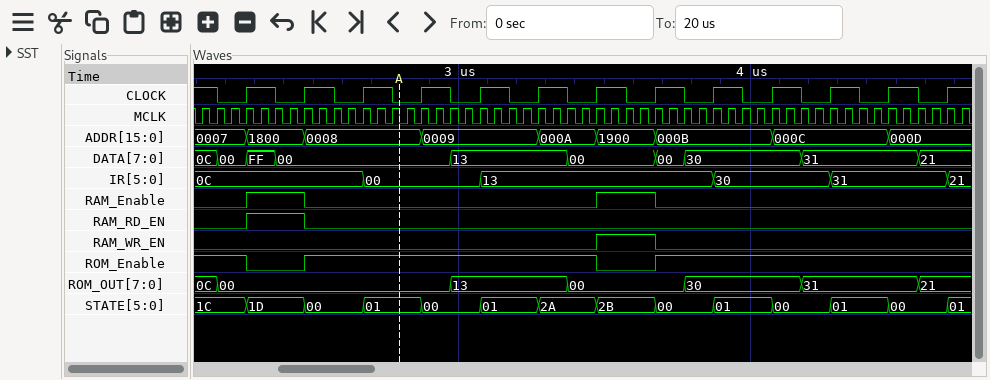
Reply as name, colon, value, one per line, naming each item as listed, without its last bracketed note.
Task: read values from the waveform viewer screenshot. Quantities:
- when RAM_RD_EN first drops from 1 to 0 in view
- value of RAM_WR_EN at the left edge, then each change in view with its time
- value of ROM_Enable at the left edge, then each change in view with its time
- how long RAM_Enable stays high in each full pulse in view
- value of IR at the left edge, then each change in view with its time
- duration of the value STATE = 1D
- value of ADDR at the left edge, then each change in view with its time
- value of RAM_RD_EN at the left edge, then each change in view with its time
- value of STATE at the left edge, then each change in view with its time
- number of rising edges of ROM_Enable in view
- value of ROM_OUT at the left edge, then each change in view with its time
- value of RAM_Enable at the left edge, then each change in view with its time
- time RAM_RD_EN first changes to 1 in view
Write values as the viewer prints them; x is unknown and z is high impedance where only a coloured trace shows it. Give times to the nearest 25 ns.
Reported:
when RAM_RD_EN first drops from 1 to 0 in view: 2475 ns
value of RAM_WR_EN at the left edge, then each change in view with its time: 0, 1 at 3475 ns, 0 at 3675 ns
value of ROM_Enable at the left edge, then each change in view with its time: 1, 0 at 2275 ns, 1 at 2475 ns, 0 at 3475 ns, 1 at 3675 ns
how long RAM_Enable stays high in each full pulse in view: 200 ns, 200 ns
value of IR at the left edge, then each change in view with its time: 0C, 00 at 2675 ns, 13 at 3075 ns, 30 at 3875 ns, 31 at 4275 ns, 21 at 4675 ns
duration of the value STATE = 1D: 200 ns
value of ADDR at the left edge, then each change in view with its time: 0007, 1800 at 2275 ns, 0008 at 2475 ns, 0009 at 2875 ns, 000A at 3275 ns, 1900 at 3475 ns, 000B at 3675 ns, 000C at 4075 ns, 000D at 4475 ns
value of RAM_RD_EN at the left edge, then each change in view with its time: 0, 1 at 2275 ns, 0 at 2475 ns
value of STATE at the left edge, then each change in view with its time: 1C, 1D at 2275 ns, 00 at 2475 ns, 01 at 2675 ns, 00 at 2875 ns, 01 at 3075 ns, 2A at 3275 ns, 2B at 3475 ns, 00 at 3675 ns, 01 at 3875 ns, 00 at 4075 ns, 01 at 4275 ns, 00 at 4475 ns, 01 at 4675 ns
number of rising edges of ROM_Enable in view: 2
value of ROM_OUT at the left edge, then each change in view with its time: 0C, 00 at 2175 ns, 13 at 2975 ns, 00 at 3375 ns, 30 at 3775 ns, 31 at 4175 ns, 21 at 4575 ns
value of RAM_Enable at the left edge, then each change in view with its time: 0, 1 at 2275 ns, 0 at 2475 ns, 1 at 3475 ns, 0 at 3675 ns
time RAM_RD_EN first changes to 1 in view: 2275 ns
